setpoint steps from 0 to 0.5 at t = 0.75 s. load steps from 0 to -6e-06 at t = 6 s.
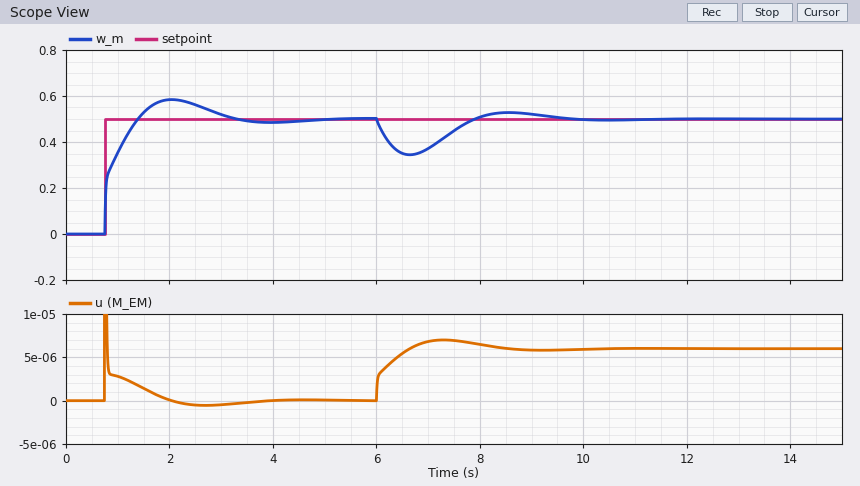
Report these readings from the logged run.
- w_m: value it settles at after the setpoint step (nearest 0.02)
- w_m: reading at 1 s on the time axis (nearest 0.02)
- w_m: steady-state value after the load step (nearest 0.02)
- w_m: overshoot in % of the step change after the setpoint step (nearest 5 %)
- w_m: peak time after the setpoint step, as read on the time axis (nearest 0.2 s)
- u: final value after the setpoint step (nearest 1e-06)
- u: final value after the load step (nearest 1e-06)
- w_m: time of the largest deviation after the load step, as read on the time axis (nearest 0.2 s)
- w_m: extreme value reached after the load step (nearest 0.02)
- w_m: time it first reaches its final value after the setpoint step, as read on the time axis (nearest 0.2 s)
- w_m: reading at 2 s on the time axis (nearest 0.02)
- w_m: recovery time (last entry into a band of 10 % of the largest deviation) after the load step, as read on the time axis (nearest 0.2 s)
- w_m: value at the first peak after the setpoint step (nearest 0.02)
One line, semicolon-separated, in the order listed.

0.50; 0.36; 0.50; 15 %; 2.0 s; 0.000000; 0.000006; 6.6 s; 0.34; 1.4 s; 0.58; 9.2 s; 0.58
